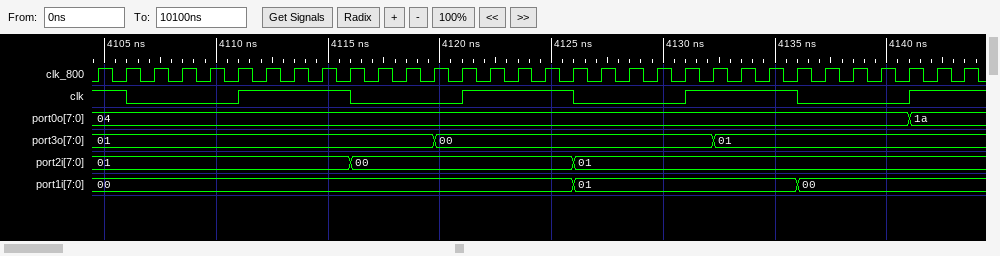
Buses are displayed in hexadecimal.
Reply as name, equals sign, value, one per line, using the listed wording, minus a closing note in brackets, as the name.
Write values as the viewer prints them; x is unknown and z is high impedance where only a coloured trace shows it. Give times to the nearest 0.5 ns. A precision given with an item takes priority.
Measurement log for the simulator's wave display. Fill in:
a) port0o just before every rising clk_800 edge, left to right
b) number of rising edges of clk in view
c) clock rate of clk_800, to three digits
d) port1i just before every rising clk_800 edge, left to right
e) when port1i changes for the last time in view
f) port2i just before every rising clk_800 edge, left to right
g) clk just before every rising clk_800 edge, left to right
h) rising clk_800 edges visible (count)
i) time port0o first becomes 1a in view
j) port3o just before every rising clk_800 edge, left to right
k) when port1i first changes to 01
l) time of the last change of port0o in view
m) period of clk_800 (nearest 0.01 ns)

port0o just before every rising clk_800 edge, left to right = 04, 04, 04, 04, 04, 04, 04, 04, 04, 04, 04, 04, 04, 04, 04, 04, 04, 04, 04, 04, 04, 04, 04, 04, 04, 04, 04, 04, 04, 04, 1a, 1a
number of rising edges of clk in view = 4
clock rate of clk_800, to three digits = 800 MHz
port1i just before every rising clk_800 edge, left to right = 00, 00, 00, 00, 00, 00, 00, 00, 00, 00, 00, 00, 00, 00, 00, 00, 00, 00, 01, 01, 01, 01, 01, 01, 01, 01, 00, 00, 00, 00, 00, 00
when port1i changes for the last time in view = 4136 ns
port2i just before every rising clk_800 edge, left to right = 01, 01, 01, 01, 01, 01, 01, 01, 01, 01, 00, 00, 00, 00, 00, 00, 00, 00, 01, 01, 01, 01, 01, 01, 01, 01, 01, 01, 01, 01, 01, 01
clk just before every rising clk_800 edge, left to right = 1 1 0 0 0 0 1 1 1 1 0 0 0 0 1 1 1 1 0 0 0 0 1 1 1 1 0 0 0 0 1 1
rising clk_800 edges visible = 32
time port0o first becomes 1a in view = 4141 ns
port3o just before every rising clk_800 edge, left to right = 01, 01, 01, 01, 01, 01, 01, 01, 01, 01, 01, 01, 01, 00, 00, 00, 00, 00, 00, 00, 00, 00, 00, 01, 01, 01, 01, 01, 01, 01, 01, 01
when port1i first changes to 01 = 4126 ns
time of the last change of port0o in view = 4141 ns
period of clk_800 = 1.25 ns
